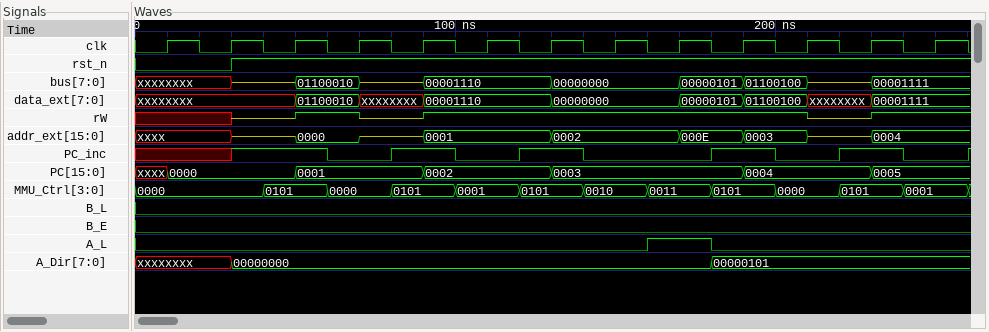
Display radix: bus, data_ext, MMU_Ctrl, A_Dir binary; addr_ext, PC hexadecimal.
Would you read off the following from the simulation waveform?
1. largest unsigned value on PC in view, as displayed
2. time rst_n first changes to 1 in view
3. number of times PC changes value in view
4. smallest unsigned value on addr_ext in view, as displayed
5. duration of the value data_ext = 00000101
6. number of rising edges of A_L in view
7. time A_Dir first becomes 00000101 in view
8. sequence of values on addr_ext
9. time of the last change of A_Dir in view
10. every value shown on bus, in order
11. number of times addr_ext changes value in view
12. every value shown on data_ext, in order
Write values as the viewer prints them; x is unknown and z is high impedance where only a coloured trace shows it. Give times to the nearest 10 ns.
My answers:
0005
30 ns
6
0000
20 ns
1
180 ns
xxxx, z, 0000, z, 0001, 0002, 000E, 0003, z, 0004
180 ns
xxxxxxxx, z, 01100010, z, 00001110, 00000000, 00000101, 01100100, z, 00001111
9
xxxxxxxx, 01100010, xxxxxxxx, 00001110, 00000000, 00000101, 01100100, xxxxxxxx, 00001111
